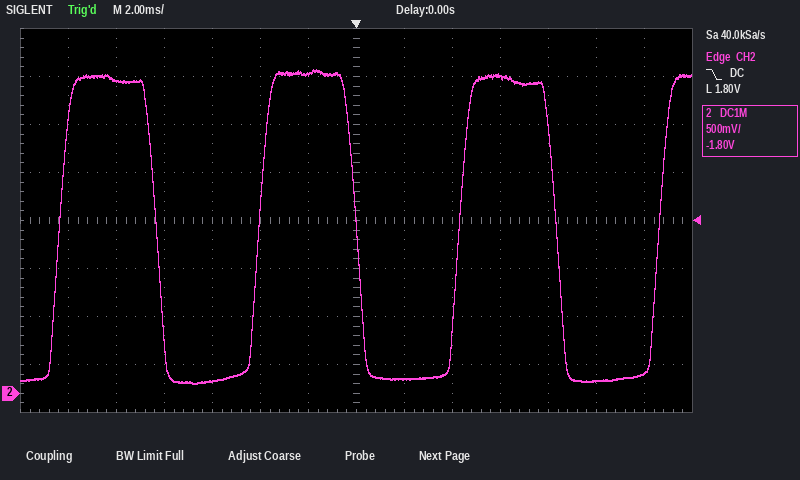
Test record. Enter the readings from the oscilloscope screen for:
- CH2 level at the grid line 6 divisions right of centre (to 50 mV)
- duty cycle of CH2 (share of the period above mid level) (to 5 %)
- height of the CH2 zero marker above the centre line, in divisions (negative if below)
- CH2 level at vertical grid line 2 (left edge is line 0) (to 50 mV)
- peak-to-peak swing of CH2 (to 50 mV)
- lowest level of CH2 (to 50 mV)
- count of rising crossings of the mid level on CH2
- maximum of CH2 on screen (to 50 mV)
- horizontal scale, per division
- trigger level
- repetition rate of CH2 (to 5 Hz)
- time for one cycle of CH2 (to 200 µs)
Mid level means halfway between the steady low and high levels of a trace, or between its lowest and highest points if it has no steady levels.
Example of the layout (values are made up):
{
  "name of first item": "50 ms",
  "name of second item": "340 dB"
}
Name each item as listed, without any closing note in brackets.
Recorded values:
{
  "CH2 level at the grid line 6 divisions right of centre": "200 mV",
  "duty cycle of CH2 (share of the period above mid level)": "50 %",
  "height of the CH2 zero marker above the centre line, in divisions": "-3.6 div",
  "CH2 level at vertical grid line 2 (left edge is line 0)": "3.25 V",
  "peak-to-peak swing of CH2": "3.25 V",
  "lowest level of CH2": "100 mV",
  "count of rising crossings of the mid level on CH2": "4",
  "maximum of CH2 on screen": "3.35 V",
  "horizontal scale, per division": "2 ms",
  "trigger level": "1.80 V",
  "repetition rate of CH2": "120 Hz",
  "time for one cycle of CH2": "8.4 ms"
}
